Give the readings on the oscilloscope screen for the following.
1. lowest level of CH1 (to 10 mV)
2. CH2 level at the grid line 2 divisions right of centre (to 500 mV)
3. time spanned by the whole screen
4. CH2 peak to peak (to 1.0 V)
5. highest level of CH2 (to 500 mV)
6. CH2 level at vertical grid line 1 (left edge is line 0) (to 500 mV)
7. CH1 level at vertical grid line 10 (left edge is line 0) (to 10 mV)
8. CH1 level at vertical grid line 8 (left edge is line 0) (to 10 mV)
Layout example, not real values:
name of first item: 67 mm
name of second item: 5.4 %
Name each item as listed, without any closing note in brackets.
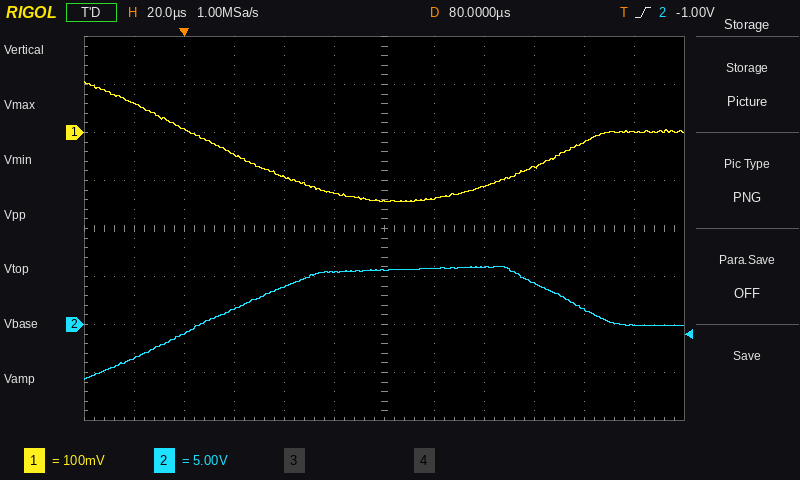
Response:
lowest level of CH1: -140 mV
CH2 level at the grid line 2 divisions right of centre: 6.0 V
time spanned by the whole screen: 240 µs
CH2 peak to peak: 12.0 V
highest level of CH2: 6.0 V
CH2 level at vertical grid line 1 (left edge is line 0): -3.5 V
CH1 level at vertical grid line 10 (left edge is line 0): -20 mV
CH1 level at vertical grid line 8 (left edge is line 0): -110 mV
